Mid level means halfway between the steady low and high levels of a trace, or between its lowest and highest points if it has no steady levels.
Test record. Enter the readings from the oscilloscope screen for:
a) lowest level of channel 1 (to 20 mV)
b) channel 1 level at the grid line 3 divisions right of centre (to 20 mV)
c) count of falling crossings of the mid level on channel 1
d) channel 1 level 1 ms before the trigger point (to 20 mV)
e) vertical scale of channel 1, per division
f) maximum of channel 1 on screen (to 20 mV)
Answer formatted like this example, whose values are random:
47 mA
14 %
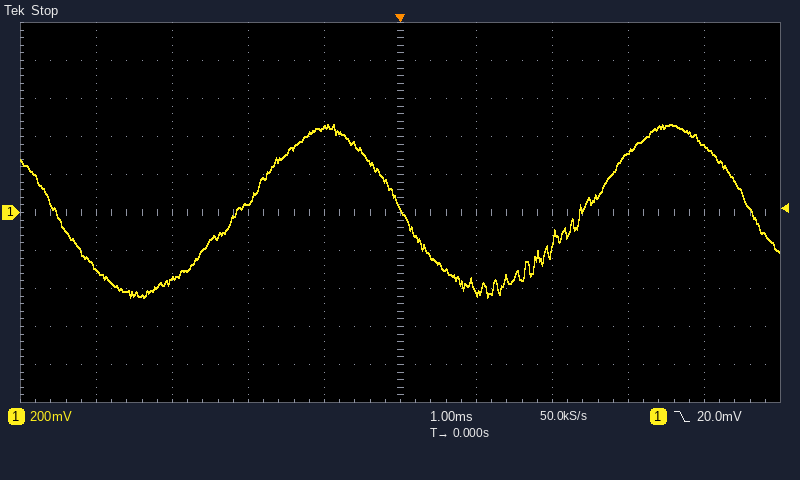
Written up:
-440 mV
320 mV
3
440 mV
200 mV
460 mV
